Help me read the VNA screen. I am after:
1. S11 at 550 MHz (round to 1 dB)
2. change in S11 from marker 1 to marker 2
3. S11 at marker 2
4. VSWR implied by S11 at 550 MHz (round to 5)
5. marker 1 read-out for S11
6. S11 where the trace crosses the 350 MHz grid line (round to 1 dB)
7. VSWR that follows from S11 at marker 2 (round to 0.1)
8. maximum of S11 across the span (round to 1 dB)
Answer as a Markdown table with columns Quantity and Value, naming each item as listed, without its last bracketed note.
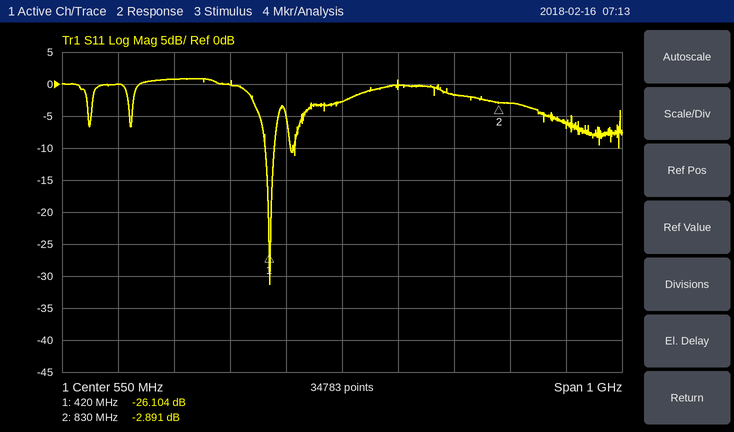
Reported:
| Quantity | Value |
|---|---|
| S11 at 550 MHz | -3 dB |
| change in S11 from marker 1 to marker 2 | 23.213 dB |
| S11 at marker 2 | -2.891 dB |
| VSWR implied by S11 at 550 MHz | 5 |
| marker 1 read-out for S11 | -26.104 dB |
| S11 where the trace crosses the 350 MHz grid line | 0 dB |
| VSWR that follows from S11 at marker 2 | 6.1 |
| maximum of S11 across the span | 1 dB |
